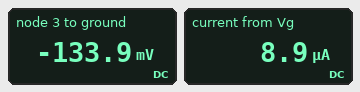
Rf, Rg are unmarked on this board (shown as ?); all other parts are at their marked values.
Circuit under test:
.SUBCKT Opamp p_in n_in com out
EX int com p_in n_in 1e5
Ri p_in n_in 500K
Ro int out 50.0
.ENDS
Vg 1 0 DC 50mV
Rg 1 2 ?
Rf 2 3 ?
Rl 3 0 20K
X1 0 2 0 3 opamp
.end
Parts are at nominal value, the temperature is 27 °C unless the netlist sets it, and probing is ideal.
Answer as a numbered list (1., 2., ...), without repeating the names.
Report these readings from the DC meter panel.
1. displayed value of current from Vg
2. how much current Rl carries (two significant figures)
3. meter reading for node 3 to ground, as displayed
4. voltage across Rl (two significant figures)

1. 8.9 µA
2. 6.7 µA
3. -133.9 mV
4. 130 mV
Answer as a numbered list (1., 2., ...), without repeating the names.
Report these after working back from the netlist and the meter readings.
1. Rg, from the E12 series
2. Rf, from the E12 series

1. 5.6 kΩ
2. 15 kΩ
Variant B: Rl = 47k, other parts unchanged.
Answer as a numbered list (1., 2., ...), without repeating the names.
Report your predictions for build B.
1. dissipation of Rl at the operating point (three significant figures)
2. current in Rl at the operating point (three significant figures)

1. 382 nW
2. 2.85 µA
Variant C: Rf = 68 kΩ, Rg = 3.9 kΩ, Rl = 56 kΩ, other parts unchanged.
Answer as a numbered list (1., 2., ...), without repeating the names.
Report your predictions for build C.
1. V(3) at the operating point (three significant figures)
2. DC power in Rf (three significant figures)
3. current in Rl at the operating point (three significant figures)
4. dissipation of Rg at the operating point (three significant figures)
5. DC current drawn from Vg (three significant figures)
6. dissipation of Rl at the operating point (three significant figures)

1. -872 mV
2. 11.2 µW
3. 15.6 µA
4. 641 nW
5. 12.8 µA
6. 13.6 µW
